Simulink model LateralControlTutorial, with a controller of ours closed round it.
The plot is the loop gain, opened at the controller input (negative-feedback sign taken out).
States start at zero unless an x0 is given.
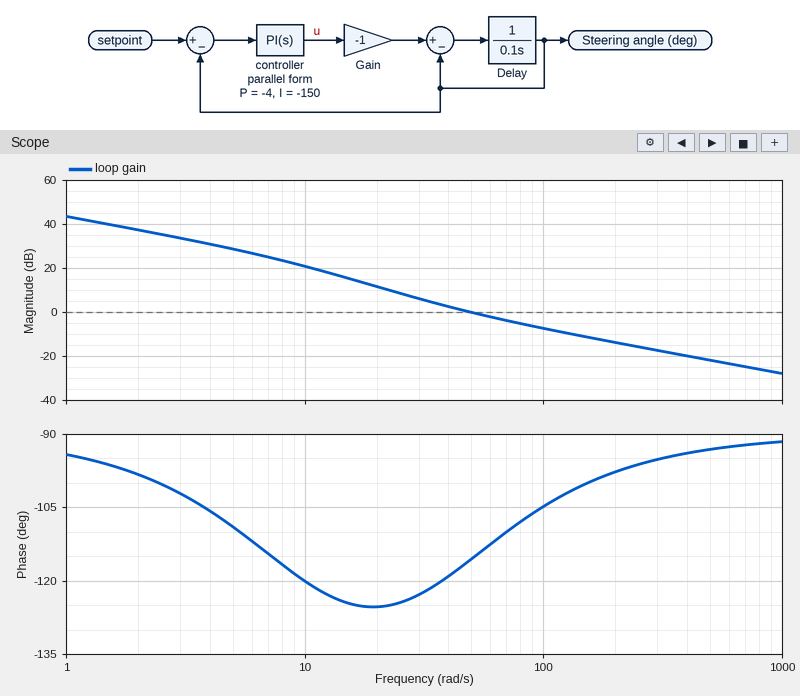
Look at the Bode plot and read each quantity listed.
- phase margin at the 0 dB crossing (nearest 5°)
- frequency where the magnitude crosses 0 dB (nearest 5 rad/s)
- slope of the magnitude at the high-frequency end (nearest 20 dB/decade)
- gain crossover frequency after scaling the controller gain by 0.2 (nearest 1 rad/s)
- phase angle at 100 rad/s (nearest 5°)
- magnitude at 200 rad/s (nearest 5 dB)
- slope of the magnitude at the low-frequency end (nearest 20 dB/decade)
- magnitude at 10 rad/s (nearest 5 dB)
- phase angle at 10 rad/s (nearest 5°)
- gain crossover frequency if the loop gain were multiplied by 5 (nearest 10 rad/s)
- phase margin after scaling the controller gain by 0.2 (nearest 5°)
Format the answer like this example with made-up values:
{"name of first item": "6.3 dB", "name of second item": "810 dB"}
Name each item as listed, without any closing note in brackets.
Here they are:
{"phase margin at the 0 dB crossing": "65°", "frequency where the magnitude crosses 0 dB": "50 rad/s", "slope of the magnitude at the high-frequency end": "-20 dB/decade", "gain crossover frequency after scaling the controller gain by 0.2": "17 rad/s", "phase angle at 100 rad/s": "-105°", "magnitude at 200 rad/s": "-15 dB", "slope of the magnitude at the low-frequency end": "-20 dB/decade", "magnitude at 10 rad/s": "20 dB", "phase angle at 10 rad/s": "-120°", "gain crossover frequency if the loop gain were multiplied by 5": "200 rad/s", "phase margin after scaling the controller gain by 0.2": "55°"}
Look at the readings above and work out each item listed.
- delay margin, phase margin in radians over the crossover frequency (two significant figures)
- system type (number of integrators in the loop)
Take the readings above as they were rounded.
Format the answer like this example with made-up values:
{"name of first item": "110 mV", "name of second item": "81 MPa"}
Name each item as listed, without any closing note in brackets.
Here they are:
{"delay margin, phase margin in radians over the crossover frequency": "0.023 s", "system type": "1"}
